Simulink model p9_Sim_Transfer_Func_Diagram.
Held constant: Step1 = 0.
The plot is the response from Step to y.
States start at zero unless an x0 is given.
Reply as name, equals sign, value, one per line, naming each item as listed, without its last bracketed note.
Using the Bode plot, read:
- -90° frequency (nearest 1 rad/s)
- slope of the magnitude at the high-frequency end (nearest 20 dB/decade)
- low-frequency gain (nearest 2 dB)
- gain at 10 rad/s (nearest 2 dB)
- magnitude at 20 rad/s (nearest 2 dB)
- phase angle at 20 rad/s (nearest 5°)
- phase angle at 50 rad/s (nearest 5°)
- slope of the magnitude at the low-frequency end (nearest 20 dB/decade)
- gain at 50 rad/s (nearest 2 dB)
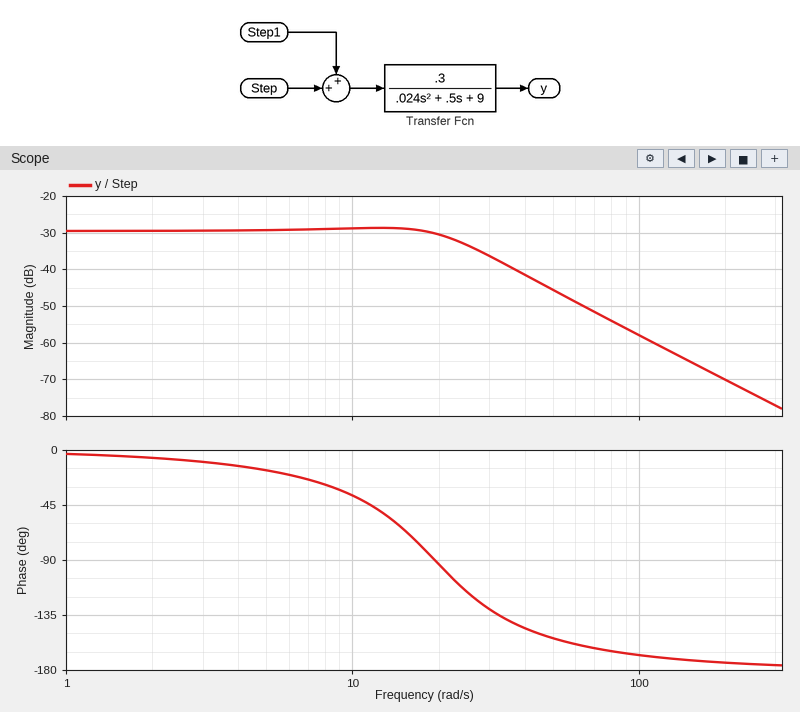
-90° frequency = 19 rad/s
slope of the magnitude at the high-frequency end = -40 dB/decade
low-frequency gain = -30 dB
gain at 10 rad/s = -28 dB
magnitude at 20 rad/s = -30 dB
phase angle at 20 rad/s = -95°
phase angle at 50 rad/s = -155°
slope of the magnitude at the low-frequency end = 0 dB/decade
gain at 50 rad/s = -46 dB
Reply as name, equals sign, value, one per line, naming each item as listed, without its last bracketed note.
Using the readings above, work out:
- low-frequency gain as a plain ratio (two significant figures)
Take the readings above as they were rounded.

low-frequency gain as a plain ratio = 0.032
